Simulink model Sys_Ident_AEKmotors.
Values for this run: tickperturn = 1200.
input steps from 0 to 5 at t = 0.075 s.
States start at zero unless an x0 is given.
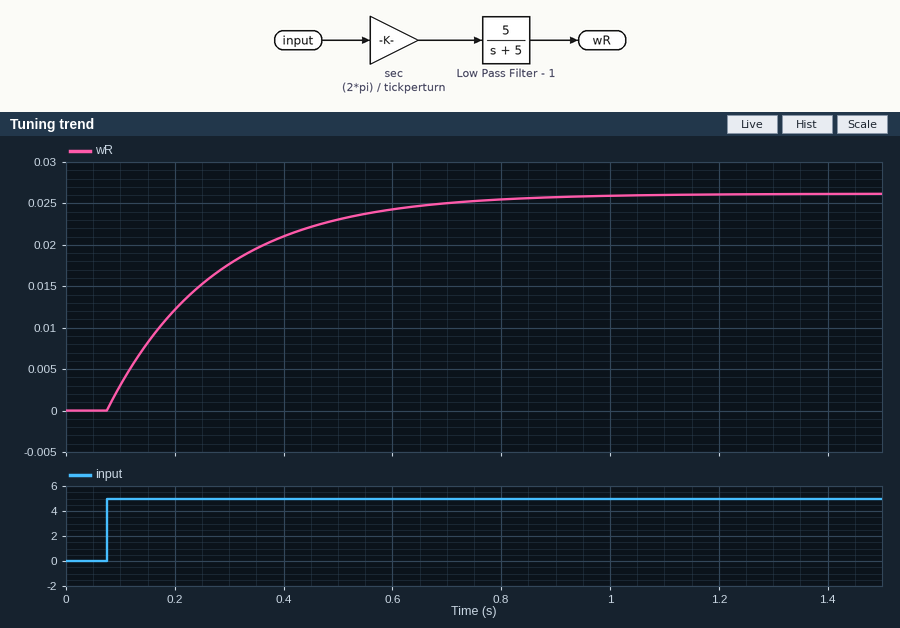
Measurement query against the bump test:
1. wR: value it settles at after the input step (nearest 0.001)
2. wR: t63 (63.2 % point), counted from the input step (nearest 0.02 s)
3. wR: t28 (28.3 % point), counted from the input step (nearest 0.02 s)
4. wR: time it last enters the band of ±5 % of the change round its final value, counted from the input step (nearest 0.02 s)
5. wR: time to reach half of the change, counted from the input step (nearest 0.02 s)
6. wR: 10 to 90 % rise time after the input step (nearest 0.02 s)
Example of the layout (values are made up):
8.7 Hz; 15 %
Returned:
0.026; 0.20 s; 0.06 s; 0.60 s; 0.14 s; 0.44 s
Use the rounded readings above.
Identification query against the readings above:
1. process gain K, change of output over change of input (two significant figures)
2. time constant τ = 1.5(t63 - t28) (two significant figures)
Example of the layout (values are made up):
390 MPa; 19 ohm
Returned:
0.0052; 0.21 s
